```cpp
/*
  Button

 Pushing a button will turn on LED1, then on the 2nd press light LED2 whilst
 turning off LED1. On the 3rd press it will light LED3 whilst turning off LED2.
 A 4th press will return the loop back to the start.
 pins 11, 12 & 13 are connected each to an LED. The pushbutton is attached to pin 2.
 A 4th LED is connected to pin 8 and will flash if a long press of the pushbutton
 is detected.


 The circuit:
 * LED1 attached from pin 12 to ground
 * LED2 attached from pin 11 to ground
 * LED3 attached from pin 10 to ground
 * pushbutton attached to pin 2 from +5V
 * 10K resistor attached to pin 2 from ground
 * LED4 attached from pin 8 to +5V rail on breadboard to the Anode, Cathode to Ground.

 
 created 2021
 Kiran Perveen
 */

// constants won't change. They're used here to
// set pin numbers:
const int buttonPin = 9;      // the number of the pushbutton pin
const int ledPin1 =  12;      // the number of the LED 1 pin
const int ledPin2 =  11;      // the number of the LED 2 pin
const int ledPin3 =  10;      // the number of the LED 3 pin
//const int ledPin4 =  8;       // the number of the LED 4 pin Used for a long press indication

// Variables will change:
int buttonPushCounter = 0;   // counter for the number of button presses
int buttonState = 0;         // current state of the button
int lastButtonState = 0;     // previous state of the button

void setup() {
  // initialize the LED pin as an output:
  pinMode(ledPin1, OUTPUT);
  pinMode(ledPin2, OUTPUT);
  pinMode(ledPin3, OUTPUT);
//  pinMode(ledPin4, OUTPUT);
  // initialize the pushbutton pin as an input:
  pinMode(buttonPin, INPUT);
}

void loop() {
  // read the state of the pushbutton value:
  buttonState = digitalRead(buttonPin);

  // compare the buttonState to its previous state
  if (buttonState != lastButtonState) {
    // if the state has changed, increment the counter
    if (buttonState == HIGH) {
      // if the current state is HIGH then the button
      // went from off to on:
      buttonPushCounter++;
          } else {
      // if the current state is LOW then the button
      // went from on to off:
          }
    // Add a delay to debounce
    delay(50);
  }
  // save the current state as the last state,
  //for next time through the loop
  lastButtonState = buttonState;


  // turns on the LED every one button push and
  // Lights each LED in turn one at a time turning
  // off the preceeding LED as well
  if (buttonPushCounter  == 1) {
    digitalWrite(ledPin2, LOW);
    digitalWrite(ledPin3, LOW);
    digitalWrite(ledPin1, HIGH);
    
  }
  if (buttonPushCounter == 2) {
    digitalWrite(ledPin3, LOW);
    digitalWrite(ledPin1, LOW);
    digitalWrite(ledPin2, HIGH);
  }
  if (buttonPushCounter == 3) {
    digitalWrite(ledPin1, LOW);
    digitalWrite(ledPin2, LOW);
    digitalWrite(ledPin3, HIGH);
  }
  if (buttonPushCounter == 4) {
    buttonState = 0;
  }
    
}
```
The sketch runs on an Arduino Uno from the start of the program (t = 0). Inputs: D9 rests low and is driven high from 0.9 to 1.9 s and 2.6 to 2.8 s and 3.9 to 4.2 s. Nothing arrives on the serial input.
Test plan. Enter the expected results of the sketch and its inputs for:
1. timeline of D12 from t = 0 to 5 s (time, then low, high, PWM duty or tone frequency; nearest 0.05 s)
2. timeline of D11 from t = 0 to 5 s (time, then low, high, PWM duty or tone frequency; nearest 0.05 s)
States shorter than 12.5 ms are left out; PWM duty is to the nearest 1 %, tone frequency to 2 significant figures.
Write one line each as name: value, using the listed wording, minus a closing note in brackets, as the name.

timeline of D12 from t = 0 to 5 s: 0 s low; 0.95 s high; 2.65 s low
timeline of D11 from t = 0 to 5 s: 0 s low; 2.65 s high; 3.95 s low
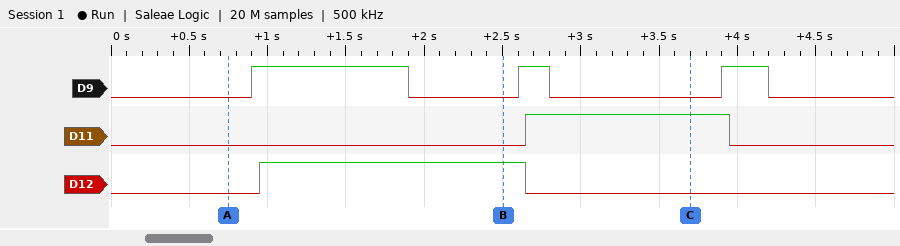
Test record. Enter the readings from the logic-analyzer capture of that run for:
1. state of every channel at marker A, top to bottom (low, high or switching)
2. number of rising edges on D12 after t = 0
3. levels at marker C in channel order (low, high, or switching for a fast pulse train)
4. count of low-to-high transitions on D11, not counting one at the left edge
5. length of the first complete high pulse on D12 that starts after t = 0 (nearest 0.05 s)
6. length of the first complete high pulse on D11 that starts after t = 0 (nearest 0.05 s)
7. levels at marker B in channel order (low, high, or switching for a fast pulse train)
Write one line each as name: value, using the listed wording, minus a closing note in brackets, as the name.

state of every channel at marker A, top to bottom: D9 low, D11 low, D12 low
number of rising edges on D12 after t = 0: 1
levels at marker C in channel order: D9 low, D11 high, D12 low
count of low-to-high transitions on D11, not counting one at the left edge: 1
length of the first complete high pulse on D12 that starts after t = 0: 1.70 s
length of the first complete high pulse on D11 that starts after t = 0: 1.30 s
levels at marker B in channel order: D9 low, D11 low, D12 high
